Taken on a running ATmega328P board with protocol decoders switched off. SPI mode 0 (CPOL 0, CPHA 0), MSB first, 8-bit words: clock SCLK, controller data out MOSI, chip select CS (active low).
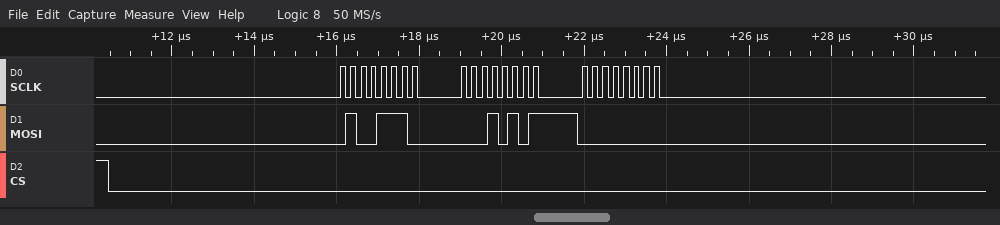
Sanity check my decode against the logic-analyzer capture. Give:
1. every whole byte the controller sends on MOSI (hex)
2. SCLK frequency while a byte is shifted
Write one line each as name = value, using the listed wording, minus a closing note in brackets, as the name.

every whole byte the controller sends on MOSI = 4E 15 00
SCLK frequency while a byte is shifted = 4 MHz
